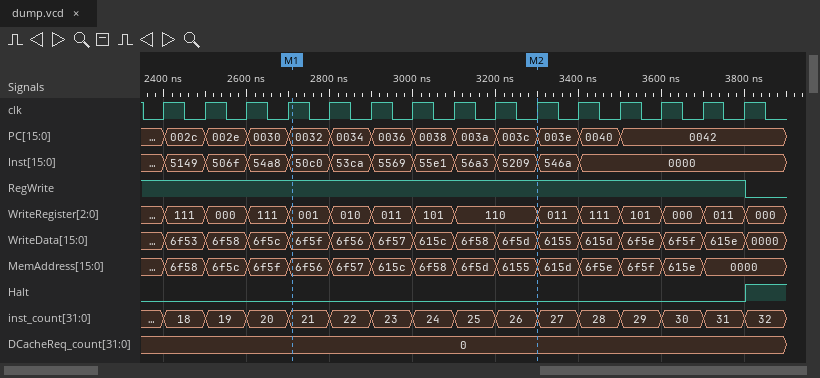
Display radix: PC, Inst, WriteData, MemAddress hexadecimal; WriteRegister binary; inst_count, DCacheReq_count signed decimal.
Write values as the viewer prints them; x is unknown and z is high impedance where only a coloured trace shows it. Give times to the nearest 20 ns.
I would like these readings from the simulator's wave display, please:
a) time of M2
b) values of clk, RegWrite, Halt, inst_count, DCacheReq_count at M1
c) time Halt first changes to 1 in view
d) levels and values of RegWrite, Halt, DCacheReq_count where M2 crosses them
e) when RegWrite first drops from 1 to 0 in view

3300 ns
clk=1, RegWrite=1, Halt=0, inst_count=21, DCacheReq_count=0
3800 ns
RegWrite=1, Halt=0, DCacheReq_count=0
3800 ns
